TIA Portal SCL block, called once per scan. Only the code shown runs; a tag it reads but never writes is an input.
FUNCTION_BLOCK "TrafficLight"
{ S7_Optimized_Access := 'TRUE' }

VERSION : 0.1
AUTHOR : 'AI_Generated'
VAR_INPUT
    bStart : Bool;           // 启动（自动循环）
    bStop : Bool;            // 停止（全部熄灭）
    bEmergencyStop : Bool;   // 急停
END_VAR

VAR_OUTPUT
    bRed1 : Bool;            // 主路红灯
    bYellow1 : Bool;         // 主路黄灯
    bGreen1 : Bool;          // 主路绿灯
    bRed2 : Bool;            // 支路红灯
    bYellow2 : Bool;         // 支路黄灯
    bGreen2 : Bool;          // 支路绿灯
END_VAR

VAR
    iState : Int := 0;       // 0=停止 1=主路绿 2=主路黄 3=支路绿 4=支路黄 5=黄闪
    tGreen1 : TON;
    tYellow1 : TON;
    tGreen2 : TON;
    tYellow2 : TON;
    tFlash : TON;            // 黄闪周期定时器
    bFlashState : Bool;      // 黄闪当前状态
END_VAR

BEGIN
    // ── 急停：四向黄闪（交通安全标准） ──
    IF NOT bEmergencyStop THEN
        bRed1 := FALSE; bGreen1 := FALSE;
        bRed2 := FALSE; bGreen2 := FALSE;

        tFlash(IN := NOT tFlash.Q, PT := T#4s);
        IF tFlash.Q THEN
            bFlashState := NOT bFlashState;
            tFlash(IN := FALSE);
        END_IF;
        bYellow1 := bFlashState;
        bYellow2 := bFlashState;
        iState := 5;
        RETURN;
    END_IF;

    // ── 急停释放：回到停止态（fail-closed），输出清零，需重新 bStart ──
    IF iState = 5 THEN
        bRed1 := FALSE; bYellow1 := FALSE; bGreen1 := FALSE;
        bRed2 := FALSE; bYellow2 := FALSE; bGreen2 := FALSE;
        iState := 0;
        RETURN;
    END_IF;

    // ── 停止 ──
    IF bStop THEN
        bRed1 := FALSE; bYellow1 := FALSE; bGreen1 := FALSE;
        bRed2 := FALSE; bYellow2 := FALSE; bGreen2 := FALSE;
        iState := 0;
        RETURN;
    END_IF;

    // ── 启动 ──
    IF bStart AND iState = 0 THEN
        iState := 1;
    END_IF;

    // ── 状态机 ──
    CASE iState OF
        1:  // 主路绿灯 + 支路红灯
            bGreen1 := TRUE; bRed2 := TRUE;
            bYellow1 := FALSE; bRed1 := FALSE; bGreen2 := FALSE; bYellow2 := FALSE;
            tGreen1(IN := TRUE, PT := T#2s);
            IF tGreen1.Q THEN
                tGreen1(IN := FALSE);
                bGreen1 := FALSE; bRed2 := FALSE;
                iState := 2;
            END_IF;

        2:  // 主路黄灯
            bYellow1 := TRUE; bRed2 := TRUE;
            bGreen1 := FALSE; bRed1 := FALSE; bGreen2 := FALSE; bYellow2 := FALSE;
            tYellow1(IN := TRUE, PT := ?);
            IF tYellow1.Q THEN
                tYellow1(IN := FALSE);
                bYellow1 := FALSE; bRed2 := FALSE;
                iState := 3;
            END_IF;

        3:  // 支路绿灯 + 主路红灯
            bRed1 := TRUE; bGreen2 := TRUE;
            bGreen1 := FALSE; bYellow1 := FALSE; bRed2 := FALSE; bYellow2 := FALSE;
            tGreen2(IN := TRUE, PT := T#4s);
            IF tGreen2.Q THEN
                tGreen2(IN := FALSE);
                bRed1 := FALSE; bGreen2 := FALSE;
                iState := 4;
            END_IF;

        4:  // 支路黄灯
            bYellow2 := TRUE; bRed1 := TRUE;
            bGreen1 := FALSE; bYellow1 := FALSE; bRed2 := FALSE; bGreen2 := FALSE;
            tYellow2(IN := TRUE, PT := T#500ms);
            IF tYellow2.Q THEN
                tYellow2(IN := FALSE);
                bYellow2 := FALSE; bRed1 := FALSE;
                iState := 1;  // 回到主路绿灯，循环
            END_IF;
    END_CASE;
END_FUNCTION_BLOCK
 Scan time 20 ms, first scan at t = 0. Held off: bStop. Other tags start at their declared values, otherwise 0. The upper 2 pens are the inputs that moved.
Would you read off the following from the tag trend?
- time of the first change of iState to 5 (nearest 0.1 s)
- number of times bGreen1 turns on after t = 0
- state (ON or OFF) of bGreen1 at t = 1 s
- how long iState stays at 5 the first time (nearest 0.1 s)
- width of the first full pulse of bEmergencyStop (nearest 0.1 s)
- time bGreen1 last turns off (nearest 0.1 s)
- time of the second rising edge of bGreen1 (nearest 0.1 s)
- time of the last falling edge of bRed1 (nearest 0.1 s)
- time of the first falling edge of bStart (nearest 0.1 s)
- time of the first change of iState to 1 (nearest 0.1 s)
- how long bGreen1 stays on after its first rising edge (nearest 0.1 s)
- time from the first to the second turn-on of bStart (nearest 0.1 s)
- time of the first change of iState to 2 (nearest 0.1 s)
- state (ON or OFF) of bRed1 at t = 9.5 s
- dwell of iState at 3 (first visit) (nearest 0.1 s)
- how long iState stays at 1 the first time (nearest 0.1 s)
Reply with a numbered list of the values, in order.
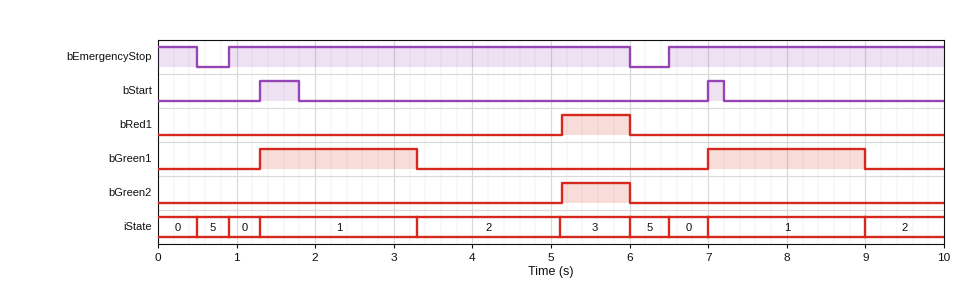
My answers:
1. 0.5 s
2. 2
3. OFF
4. 0.4 s
5. 5.1 s
6. 9.0 s
7. 7.0 s
8. 6.0 s
9. 1.8 s
10. 1.3 s
11. 2.0 s
12. 5.7 s
13. 3.3 s
14. OFF
15. 0.9 s
16. 2.0 s
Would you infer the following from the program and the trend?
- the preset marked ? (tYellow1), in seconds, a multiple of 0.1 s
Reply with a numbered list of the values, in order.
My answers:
1. 1.8 s
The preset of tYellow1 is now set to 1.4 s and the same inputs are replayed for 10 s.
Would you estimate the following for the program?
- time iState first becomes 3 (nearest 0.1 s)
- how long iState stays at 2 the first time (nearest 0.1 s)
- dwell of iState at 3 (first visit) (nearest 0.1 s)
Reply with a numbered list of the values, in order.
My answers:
1. 4.7 s
2. 1.4 s
3. 1.3 s
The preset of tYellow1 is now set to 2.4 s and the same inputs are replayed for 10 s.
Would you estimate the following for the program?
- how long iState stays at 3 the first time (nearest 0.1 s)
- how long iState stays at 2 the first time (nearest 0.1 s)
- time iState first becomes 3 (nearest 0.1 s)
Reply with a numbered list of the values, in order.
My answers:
1. 0.3 s
2. 2.4 s
3. 5.7 s
